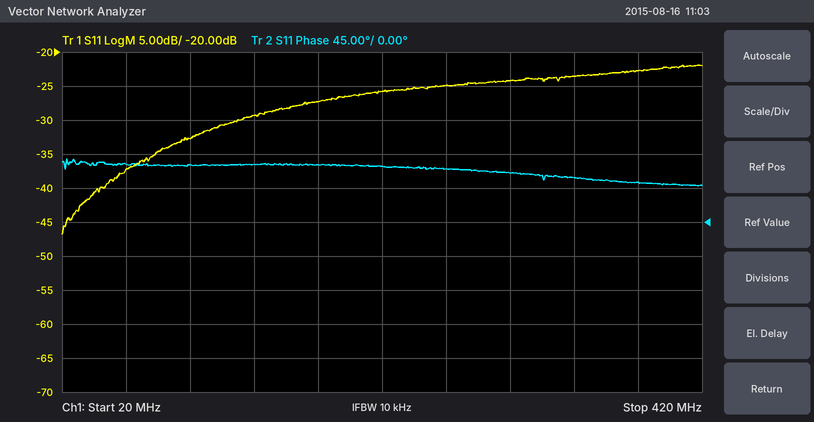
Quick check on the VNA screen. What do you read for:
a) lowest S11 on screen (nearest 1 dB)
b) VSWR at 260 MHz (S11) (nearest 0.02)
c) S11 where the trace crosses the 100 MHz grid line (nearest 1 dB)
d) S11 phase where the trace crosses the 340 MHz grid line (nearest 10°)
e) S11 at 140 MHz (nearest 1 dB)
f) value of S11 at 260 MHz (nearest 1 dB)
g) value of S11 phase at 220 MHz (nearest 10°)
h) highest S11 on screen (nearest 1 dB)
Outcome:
-47 dB
1.12
-33 dB
60°
-29 dB
-25 dB
70°
-22 dB
